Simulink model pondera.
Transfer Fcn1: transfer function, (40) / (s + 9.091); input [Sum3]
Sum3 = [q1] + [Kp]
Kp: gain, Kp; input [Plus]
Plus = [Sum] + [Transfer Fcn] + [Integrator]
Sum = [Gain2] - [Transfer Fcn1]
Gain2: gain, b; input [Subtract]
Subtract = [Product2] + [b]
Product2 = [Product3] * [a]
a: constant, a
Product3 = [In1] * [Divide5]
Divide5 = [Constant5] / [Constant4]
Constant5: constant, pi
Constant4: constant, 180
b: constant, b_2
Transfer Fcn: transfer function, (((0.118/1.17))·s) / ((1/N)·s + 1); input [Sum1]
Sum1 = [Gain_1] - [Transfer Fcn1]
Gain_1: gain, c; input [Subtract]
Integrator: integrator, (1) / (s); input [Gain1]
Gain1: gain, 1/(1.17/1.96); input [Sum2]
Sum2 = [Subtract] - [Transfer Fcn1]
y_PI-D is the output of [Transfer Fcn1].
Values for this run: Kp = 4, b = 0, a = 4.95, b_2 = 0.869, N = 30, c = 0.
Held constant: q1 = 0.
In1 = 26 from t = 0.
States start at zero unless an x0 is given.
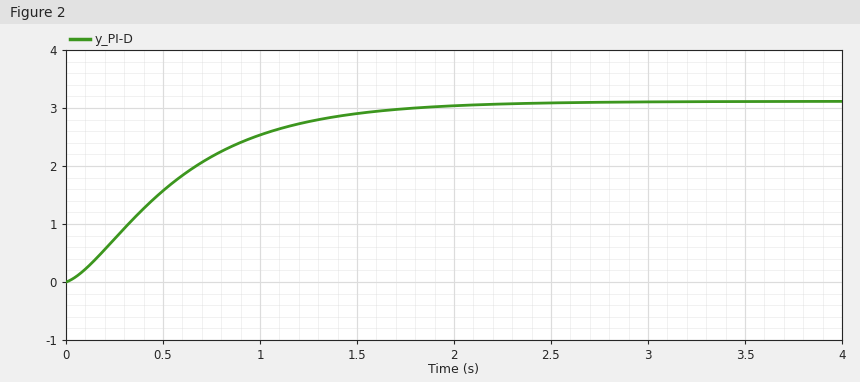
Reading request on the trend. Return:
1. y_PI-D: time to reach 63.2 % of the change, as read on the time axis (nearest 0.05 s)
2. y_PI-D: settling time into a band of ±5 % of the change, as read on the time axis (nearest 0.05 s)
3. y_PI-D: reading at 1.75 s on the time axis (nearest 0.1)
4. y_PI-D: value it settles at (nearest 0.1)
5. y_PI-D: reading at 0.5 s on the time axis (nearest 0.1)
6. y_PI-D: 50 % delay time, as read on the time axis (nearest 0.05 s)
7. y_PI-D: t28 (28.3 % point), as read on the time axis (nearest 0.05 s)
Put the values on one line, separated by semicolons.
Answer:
0.65 s; 1.65 s; 3.0; 3.1; 1.6; 0.50 s; 0.30 s
